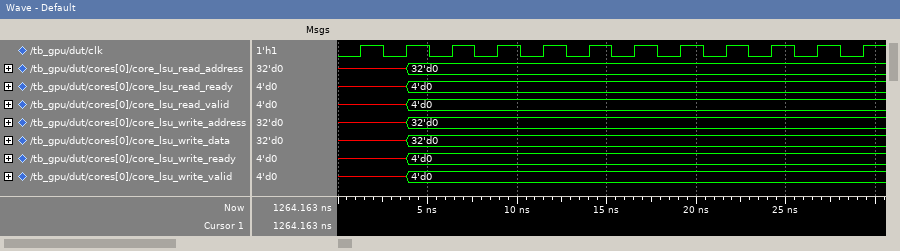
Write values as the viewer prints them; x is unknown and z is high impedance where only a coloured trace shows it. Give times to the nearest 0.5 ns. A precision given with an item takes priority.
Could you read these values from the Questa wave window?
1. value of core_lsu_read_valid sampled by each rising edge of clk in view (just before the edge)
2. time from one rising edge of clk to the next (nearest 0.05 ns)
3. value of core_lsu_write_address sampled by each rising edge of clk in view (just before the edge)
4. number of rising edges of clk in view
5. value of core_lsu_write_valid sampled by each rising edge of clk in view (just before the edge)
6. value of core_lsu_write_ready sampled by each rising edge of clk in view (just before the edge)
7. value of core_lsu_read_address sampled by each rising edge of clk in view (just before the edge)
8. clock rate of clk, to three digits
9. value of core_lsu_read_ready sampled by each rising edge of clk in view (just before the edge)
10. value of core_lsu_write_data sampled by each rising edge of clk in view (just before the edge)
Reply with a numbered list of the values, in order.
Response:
1. x, x, 4'd0, 4'd0, 4'd0, 4'd0, 4'd0, 4'd0, 4'd0, 4'd0, 4'd0, 4'd0
2. 2.55 ns
3. x, x, 32'd0, 32'd0, 32'd0, 32'd0, 32'd0, 32'd0, 32'd0, 32'd0, 32'd0, 32'd0
4. 12
5. x, x, 4'd0, 4'd0, 4'd0, 4'd0, 4'd0, 4'd0, 4'd0, 4'd0, 4'd0, 4'd0
6. x, x, 4'd0, 4'd0, 4'd0, 4'd0, 4'd0, 4'd0, 4'd0, 4'd0, 4'd0, 4'd0
7. x, x, 32'd0, 32'd0, 32'd0, 32'd0, 32'd0, 32'd0, 32'd0, 32'd0, 32'd0, 32'd0
8. 392 MHz
9. x, x, 4'd0, 4'd0, 4'd0, 4'd0, 4'd0, 4'd0, 4'd0, 4'd0, 4'd0, 4'd0
10. x, x, 32'd0, 32'd0, 32'd0, 32'd0, 32'd0, 32'd0, 32'd0, 32'd0, 32'd0, 32'd0
